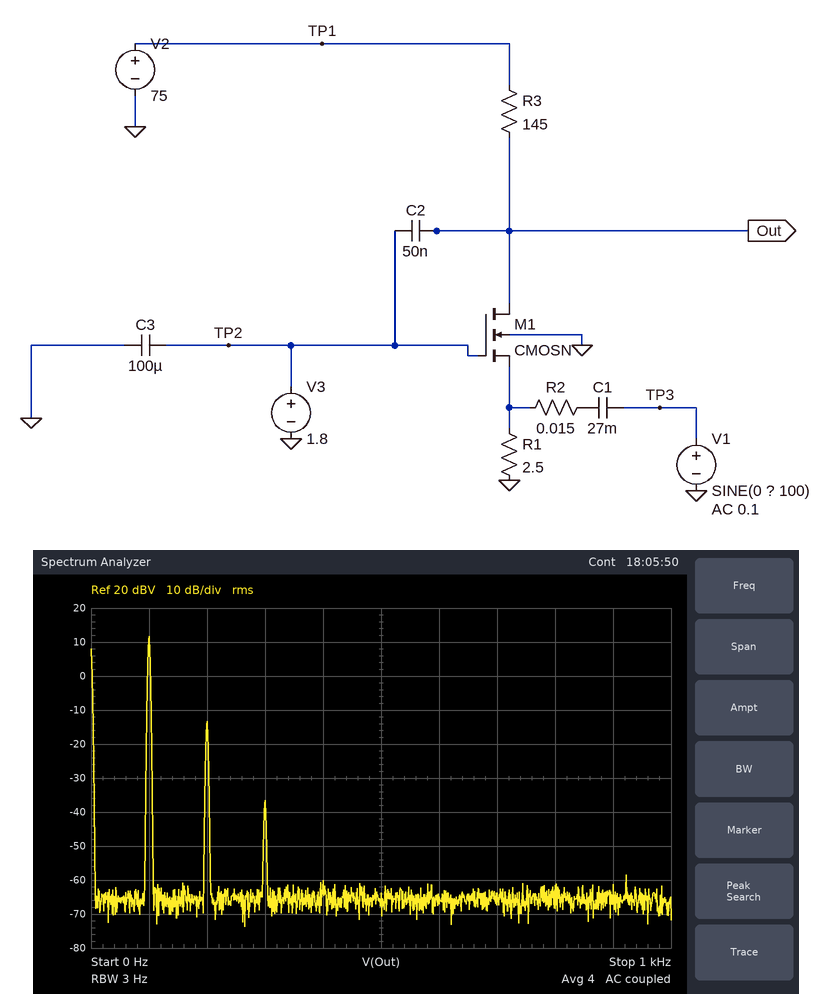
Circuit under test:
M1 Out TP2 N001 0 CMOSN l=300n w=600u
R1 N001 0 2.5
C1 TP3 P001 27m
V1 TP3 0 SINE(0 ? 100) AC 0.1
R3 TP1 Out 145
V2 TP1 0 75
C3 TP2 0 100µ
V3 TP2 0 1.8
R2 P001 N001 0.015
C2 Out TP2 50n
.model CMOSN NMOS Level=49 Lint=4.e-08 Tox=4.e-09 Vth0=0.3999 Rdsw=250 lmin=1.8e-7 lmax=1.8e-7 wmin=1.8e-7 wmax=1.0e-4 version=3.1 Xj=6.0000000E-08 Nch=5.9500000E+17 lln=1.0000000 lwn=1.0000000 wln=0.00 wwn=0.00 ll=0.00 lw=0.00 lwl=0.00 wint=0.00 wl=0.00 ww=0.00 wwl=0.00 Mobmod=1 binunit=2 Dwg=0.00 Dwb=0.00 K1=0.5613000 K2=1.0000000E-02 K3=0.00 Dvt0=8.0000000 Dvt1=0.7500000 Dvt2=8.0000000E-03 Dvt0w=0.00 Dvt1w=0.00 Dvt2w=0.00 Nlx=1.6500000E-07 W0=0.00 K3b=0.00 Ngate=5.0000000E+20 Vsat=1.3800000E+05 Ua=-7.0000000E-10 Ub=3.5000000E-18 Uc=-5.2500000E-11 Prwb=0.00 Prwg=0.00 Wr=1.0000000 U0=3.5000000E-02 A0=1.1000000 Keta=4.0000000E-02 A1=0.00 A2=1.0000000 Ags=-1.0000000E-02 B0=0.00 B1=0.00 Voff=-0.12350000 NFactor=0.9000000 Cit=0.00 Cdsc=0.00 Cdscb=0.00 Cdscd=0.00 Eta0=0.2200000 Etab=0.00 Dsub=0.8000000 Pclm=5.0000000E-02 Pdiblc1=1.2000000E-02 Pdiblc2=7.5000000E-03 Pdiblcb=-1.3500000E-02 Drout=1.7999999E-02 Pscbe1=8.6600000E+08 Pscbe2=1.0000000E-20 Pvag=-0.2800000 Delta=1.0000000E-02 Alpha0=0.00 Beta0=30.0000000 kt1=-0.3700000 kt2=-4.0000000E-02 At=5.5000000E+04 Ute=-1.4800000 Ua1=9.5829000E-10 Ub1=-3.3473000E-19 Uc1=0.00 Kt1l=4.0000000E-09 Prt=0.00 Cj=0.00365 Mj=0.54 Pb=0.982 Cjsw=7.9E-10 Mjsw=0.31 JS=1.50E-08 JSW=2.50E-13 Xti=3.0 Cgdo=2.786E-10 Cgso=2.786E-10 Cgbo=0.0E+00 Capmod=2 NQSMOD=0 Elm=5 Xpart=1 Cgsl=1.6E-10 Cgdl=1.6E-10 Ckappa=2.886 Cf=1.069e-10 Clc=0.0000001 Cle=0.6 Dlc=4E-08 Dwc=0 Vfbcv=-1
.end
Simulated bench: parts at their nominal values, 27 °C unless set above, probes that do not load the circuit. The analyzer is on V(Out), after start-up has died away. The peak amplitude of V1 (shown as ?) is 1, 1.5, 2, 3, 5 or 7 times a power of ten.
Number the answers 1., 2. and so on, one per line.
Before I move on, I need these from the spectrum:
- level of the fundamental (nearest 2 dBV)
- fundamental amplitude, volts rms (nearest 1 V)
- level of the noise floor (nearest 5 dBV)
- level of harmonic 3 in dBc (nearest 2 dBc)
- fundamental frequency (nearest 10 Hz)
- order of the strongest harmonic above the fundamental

1. 12 dBV
2. 4 V
3. -65 dBV
4. -48 dBc
5. 100 Hz
6. 2
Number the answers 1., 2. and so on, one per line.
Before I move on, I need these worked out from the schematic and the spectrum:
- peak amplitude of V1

1. 150 mV
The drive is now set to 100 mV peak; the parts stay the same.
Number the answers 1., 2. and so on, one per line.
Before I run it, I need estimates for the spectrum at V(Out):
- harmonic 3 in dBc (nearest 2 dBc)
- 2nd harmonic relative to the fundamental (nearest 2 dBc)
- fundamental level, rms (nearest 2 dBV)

1. -56 dBc
2. -28 dBc
3. 8 dBV
